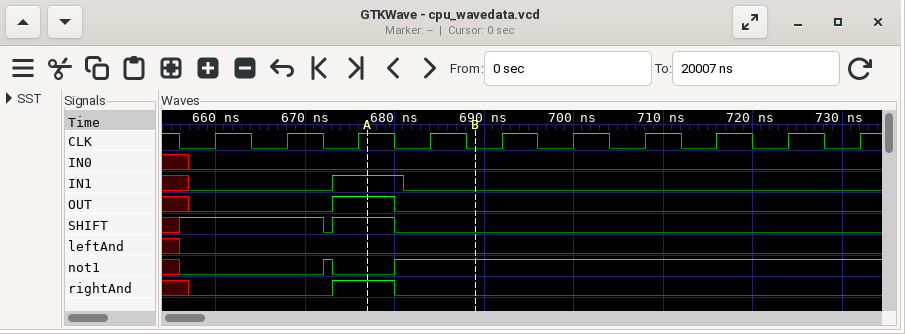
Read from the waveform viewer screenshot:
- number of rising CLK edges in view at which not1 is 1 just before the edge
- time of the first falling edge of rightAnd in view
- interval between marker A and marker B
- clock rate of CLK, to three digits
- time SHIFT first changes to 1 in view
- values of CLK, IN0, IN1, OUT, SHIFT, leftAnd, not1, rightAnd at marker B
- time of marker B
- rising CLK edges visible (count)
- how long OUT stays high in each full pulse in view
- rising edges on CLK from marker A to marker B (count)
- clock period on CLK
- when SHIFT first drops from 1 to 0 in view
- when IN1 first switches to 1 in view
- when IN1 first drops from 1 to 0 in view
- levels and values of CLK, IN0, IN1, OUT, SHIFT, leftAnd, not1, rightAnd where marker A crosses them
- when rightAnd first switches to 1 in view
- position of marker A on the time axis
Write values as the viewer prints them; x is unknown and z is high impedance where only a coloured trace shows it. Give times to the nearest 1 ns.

7
680 ns
12 ns
125 MHz
656 ns
CLK=0, IN0=0, IN1=0, OUT=0, SHIFT=0, leftAnd=0, not1=1, rightAnd=0
689 ns
10
7 ns
1
8 ns
672 ns
673 ns
681 ns
CLK=1, IN0=0, IN1=1, OUT=1, SHIFT=1, leftAnd=0, not1=0, rightAnd=1
673 ns
677 ns
